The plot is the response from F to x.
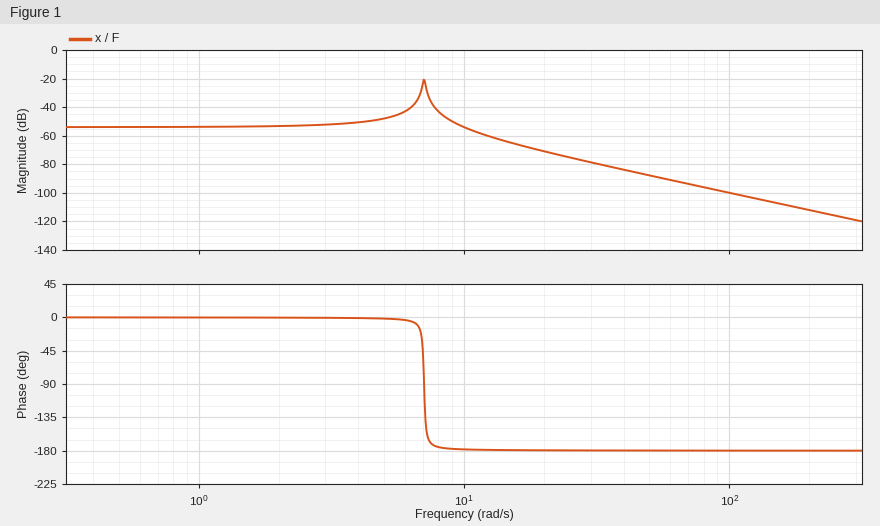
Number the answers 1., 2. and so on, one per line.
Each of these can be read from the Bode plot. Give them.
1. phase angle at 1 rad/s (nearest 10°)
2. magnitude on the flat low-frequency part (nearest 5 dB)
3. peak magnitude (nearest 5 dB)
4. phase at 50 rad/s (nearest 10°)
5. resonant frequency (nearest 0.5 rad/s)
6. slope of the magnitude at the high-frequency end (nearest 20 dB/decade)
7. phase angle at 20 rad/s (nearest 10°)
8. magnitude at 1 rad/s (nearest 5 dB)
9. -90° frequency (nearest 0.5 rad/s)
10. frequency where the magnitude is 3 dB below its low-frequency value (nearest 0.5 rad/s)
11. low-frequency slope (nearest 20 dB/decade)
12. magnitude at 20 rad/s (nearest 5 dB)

1. 0°
2. -55 dB
3. -20 dB
4. -180°
5. 7.0 rad/s
6. -40 dB/decade
7. -180°
8. -55 dB
9. 7.0 rad/s
10. 11.0 rad/s
11. 0 dB/decade
12. -70 dB
